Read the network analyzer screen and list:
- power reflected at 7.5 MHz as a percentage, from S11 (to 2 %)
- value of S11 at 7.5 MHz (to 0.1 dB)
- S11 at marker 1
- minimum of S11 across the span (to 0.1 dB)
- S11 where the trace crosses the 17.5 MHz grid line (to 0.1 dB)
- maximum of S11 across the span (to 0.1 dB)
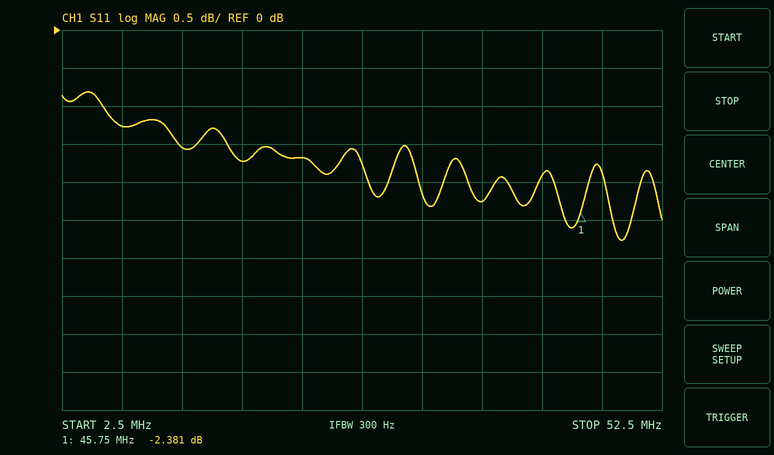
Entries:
74 %
-1.3 dB
-2.381 dB
-2.8 dB
-1.7 dB
-0.8 dB
